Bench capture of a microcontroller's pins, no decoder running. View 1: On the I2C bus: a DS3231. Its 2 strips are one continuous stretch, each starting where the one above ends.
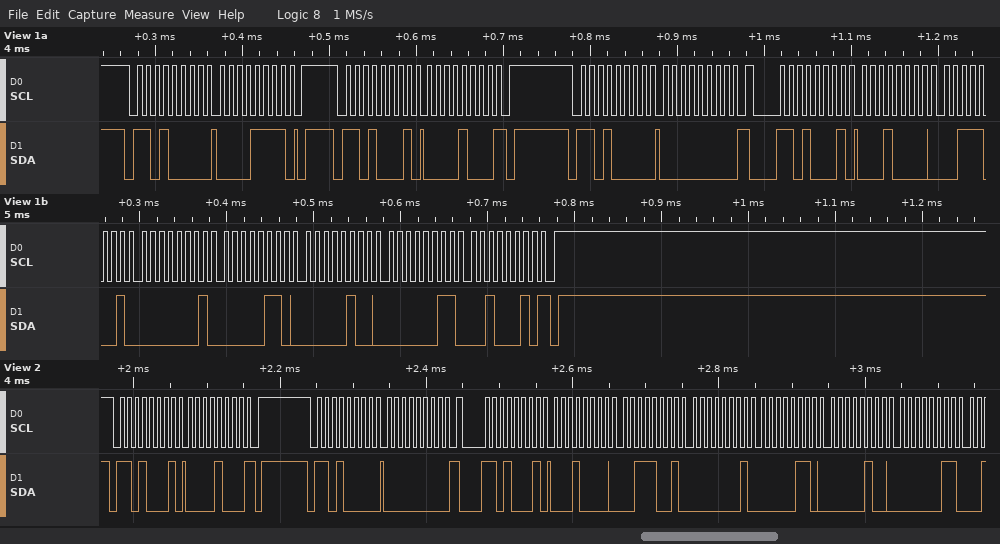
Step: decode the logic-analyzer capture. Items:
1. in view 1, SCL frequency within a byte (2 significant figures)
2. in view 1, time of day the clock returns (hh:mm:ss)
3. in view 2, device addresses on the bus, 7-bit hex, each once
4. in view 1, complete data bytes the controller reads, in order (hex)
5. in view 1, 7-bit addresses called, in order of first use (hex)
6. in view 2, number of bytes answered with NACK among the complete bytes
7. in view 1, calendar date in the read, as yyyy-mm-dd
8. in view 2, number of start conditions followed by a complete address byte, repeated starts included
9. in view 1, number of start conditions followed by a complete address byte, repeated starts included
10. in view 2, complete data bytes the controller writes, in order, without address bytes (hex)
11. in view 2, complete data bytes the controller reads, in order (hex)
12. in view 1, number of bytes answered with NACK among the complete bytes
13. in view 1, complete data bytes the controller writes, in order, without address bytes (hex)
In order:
100 kHz
01:39:10
0x68
08 10 39 01 06 04 03 22
0x68
1
2022-03-04
3
4
00
08 10 39 01 06 04 03
2
0F 00
